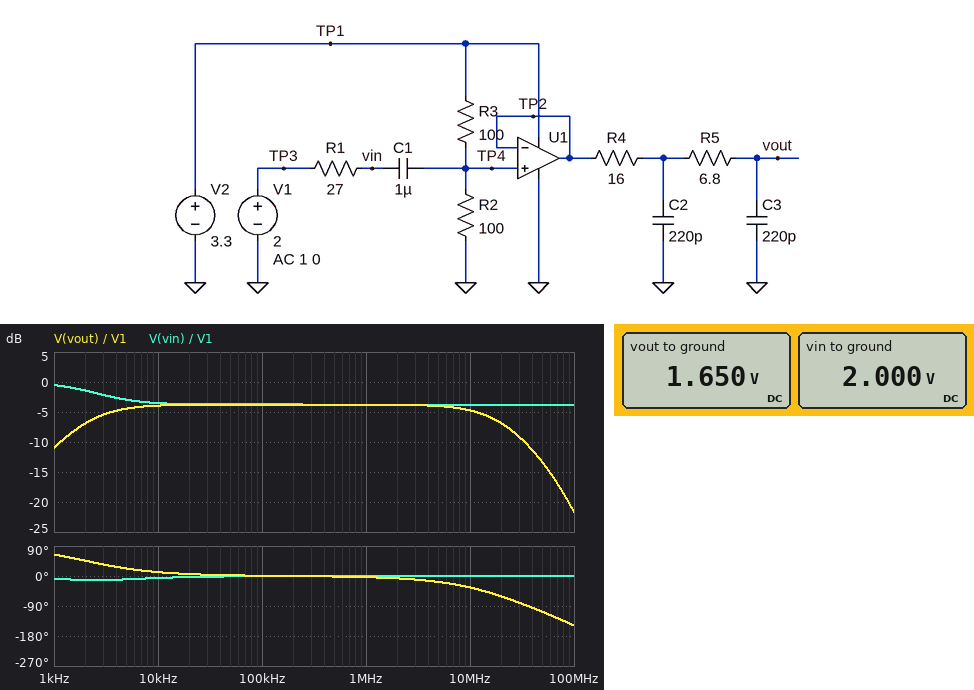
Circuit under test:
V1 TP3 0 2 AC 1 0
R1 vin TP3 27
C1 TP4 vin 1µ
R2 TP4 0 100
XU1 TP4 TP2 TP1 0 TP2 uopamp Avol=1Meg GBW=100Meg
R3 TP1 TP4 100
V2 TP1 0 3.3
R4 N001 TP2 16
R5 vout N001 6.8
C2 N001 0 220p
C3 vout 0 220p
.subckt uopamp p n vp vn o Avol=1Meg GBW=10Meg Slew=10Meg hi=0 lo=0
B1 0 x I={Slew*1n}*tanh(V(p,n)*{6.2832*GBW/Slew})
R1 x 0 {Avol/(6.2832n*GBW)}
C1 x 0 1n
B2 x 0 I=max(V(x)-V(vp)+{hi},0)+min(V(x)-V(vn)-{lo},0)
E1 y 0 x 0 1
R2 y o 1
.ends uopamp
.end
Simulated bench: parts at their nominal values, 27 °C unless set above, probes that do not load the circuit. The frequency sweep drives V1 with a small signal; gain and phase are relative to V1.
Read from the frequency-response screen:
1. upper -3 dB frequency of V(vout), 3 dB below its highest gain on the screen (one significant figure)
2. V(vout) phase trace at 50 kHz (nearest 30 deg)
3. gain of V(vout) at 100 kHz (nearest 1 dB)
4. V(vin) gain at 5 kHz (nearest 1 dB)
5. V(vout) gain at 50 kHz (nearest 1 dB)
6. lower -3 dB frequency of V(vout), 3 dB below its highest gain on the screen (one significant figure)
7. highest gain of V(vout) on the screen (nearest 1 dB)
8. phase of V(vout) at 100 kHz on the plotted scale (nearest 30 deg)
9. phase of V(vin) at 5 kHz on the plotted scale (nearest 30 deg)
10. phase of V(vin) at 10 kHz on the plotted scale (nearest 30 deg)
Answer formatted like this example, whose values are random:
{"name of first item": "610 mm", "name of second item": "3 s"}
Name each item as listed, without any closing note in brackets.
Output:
{"upper -3 dB frequency of V(vout), 3 dB below its highest gain on the screen": "20 MHz", "V(vout) phase trace at 50 kHz": "0 deg", "gain of V(vout) at 100 kHz": "-4 dB", "V(vin) gain at 5 kHz": "-3 dB", "V(vout) gain at 50 kHz": "-4 dB", "lower -3 dB frequency of V(vout), 3 dB below its highest gain on the screen": "2 kHz", "highest gain of V(vout) on the screen": "-4 dB", "phase of V(vout) at 100 kHz on the plotted scale": "0 deg", "phase of V(vin) at 5 kHz on the plotted scale": "0 deg", "phase of V(vin) at 10 kHz on the plotted scale": "0 deg"}
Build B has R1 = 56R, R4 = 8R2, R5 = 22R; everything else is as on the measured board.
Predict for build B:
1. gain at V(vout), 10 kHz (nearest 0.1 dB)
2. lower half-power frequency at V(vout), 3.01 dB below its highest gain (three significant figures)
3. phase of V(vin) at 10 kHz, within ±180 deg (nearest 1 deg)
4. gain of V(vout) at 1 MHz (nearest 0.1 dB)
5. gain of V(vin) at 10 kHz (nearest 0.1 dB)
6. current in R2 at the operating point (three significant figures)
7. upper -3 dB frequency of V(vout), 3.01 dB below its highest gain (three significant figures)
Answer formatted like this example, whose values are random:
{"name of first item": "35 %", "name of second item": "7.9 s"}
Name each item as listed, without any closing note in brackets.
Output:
{"gain at V(vout), 10 kHz": "-6.6 dB", "lower half-power frequency at V(vout), 3.01 dB below its highest gain": "1.50 kHz", "phase of V(vin) at 10 kHz, within ±180 deg": "-9 deg", "gain of V(vout) at 1 MHz": "-6.5 dB", "gain of V(vin) at 10 kHz": "-6.2 dB", "current in R2 at the operating point": "16.5 mA", "upper -3 dB frequency of V(vout), 3.01 dB below its highest gain": "20.8 MHz"}
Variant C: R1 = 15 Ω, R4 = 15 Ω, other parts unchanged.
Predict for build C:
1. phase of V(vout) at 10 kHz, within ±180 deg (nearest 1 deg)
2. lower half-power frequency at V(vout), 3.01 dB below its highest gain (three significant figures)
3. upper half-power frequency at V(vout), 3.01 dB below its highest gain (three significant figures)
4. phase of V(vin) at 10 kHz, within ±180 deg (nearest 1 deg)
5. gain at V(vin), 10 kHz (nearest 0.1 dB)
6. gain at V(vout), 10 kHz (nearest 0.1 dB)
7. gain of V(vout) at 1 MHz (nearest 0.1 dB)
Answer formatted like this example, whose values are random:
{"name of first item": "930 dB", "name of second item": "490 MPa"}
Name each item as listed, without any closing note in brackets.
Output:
{"phase of V(vout) at 10 kHz, within ±180 deg": "14 deg", "lower half-power frequency at V(vout), 3.01 dB below its highest gain": "2.45 kHz", "upper half-power frequency at V(vout), 3.01 dB below its highest gain": "20.6 MHz", "phase of V(vin) at 10 kHz, within ±180 deg": "-4 deg", "gain at V(vin), 10 kHz": "-2.1 dB", "gain at V(vout), 10 kHz": "-2.5 dB", "gain of V(vout) at 1 MHz": "-2.3 dB"}
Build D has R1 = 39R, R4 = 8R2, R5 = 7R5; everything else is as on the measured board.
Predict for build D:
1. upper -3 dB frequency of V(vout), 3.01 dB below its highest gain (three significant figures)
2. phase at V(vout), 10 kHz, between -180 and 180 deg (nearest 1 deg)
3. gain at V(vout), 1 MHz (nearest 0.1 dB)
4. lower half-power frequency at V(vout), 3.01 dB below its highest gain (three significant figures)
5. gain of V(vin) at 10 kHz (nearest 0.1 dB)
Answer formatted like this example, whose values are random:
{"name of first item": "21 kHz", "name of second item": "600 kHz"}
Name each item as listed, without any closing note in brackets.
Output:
{"upper -3 dB frequency of V(vout), 3.01 dB below its highest gain": "31.4 MHz", "phase at V(vout), 10 kHz, between -180 and 180 deg": "10 deg", "gain at V(vout), 1 MHz": "-5.0 dB", "lower half-power frequency at V(vout), 3.01 dB below its highest gain": "1.79 kHz", "gain of V(vin) at 10 kHz": "-4.7 dB"}
